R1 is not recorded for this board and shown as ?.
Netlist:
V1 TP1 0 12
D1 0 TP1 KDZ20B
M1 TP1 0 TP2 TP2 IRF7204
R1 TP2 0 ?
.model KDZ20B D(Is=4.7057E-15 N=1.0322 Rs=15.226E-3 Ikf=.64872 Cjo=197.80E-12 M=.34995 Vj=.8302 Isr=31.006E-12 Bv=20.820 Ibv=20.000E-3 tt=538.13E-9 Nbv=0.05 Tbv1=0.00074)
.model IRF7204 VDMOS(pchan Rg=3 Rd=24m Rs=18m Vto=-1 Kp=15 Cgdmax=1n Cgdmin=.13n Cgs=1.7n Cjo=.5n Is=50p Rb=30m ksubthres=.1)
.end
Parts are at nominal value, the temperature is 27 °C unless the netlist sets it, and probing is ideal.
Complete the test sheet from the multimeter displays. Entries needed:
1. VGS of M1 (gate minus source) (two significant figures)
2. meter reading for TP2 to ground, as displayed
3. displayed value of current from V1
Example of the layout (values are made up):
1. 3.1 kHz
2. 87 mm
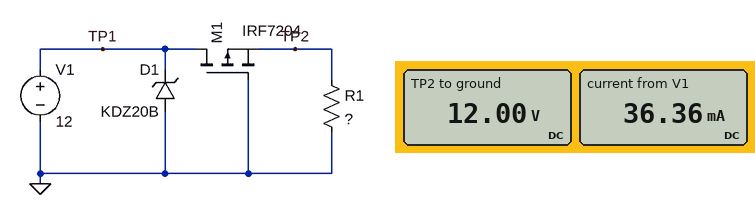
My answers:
1. -12 V
2. 12.00 V
3. 36.36 mA
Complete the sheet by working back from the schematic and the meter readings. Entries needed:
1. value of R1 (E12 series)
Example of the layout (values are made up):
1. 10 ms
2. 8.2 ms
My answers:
1. 330 Ω
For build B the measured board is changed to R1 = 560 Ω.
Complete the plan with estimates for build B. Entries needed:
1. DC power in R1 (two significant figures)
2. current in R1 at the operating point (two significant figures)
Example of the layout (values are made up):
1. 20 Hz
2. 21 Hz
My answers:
1. 260 mW
2. 21 mA
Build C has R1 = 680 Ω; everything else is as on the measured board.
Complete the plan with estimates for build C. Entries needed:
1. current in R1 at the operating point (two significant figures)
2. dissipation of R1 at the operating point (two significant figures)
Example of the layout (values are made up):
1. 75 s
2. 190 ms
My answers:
1. 18 mA
2. 210 mW
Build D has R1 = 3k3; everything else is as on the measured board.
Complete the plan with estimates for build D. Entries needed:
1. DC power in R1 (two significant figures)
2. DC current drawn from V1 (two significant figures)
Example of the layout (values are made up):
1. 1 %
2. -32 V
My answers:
1. 44 mW
2. 3.6 mA
